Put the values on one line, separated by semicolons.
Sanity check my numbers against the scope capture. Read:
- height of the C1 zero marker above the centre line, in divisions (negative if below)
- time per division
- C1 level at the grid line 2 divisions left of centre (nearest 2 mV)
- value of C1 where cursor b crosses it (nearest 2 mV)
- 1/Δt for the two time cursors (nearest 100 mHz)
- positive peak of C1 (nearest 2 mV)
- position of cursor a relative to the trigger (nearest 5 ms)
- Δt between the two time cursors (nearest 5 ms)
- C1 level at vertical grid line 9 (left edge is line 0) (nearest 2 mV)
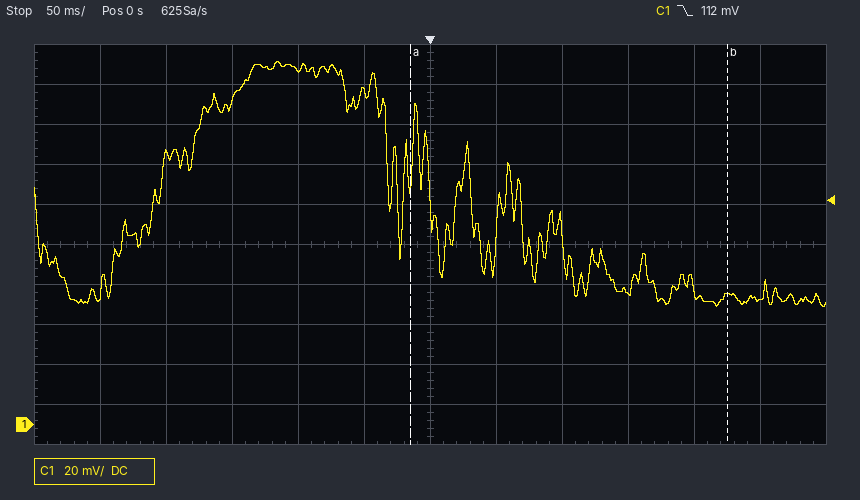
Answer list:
-4.5 div; 50 ms; 178 mV; 64 mV; 4.2 Hz; 182 mV; -15 ms; 240 ms; 66 mV
